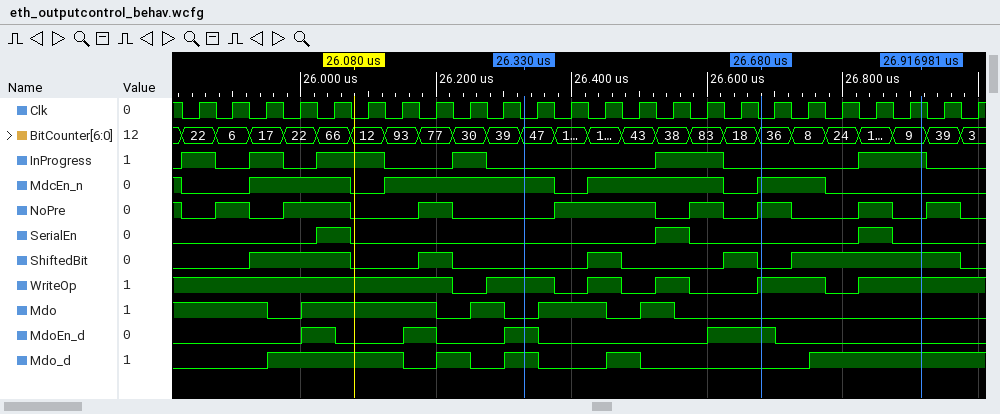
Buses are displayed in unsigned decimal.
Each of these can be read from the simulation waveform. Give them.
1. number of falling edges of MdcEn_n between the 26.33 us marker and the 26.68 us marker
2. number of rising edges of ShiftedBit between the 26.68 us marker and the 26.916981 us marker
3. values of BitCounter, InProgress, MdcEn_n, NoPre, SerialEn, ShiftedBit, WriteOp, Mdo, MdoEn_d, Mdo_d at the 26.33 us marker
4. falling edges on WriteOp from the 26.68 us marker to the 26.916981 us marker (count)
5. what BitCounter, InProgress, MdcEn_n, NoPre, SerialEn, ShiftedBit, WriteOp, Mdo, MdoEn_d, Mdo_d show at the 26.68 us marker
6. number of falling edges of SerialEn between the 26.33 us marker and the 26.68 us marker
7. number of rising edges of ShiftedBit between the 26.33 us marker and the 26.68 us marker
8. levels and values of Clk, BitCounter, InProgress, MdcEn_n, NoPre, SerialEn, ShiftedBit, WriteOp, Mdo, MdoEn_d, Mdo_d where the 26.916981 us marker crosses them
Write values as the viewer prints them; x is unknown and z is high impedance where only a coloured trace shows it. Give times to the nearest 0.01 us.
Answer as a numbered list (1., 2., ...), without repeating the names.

1. 2
2. 1
3. BitCounter=47, InProgress=0, MdcEn_n=1, NoPre=0, SerialEn=0, ShiftedBit=0, WriteOp=1, Mdo=0, MdoEn_d=1, Mdo_d=1
4. 1
5. BitCounter=36, InProgress=0, MdcEn_n=1, NoPre=1, SerialEn=0, ShiftedBit=0, WriteOp=1, Mdo=0, MdoEn_d=1, Mdo_d=0
6. 1
7. 2
8. Clk=1, BitCounter=9, InProgress=1, MdcEn_n=0, NoPre=0, SerialEn=0, ShiftedBit=1, WriteOp=1, Mdo=0, MdoEn_d=0, Mdo_d=1
